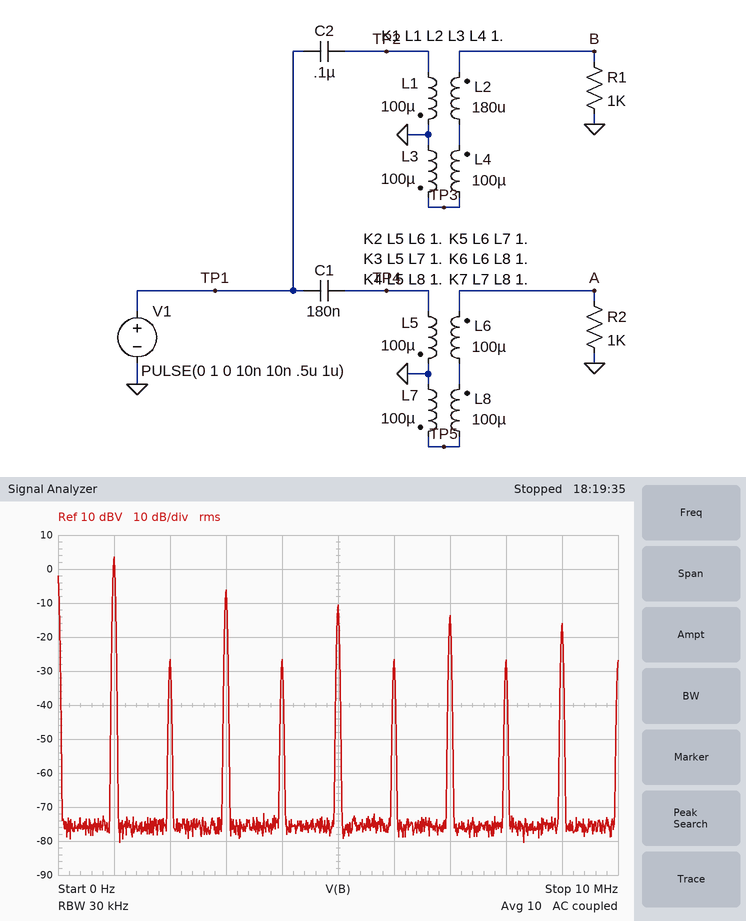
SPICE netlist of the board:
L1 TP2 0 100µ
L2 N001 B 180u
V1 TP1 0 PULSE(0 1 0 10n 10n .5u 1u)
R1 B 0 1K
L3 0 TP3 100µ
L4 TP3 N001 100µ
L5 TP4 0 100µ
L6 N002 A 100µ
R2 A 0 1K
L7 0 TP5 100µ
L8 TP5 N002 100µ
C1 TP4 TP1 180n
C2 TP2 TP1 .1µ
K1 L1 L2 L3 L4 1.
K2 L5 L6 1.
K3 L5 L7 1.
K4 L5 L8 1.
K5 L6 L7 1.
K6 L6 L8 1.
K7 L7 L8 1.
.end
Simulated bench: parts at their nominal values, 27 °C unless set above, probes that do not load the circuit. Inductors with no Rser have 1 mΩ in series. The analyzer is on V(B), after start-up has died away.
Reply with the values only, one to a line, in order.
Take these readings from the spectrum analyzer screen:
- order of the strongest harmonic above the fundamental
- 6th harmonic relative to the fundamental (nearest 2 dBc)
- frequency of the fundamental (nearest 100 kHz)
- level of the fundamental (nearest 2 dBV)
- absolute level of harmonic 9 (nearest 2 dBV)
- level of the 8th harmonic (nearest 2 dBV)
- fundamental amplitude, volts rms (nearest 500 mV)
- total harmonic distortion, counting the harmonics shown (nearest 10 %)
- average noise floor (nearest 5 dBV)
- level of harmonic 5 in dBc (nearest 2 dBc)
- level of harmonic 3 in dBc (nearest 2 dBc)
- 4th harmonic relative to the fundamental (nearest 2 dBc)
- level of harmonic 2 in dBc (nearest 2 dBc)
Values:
3
-30 dBc
1.0 MHz
4 dBV
-16 dBV
-26 dBV
1.5 V
40 %
-75 dBV
-14 dBc
-10 dBc
-30 dBc
-30 dBc
